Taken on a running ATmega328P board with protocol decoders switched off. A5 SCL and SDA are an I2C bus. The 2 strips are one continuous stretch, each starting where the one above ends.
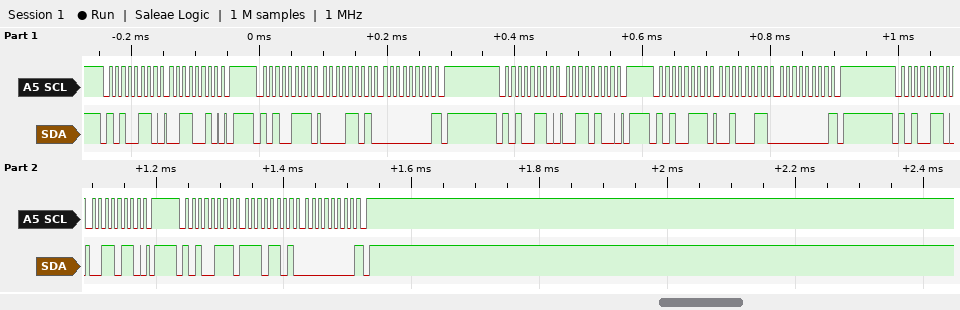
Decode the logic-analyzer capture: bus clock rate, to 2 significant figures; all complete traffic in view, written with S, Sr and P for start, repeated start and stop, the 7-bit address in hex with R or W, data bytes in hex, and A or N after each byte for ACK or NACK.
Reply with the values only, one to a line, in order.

100 kHz
S 53W A 32 A P S 53R A 0D A 00 N P S 53W A 34 A P S 53R A 23 A 00 N P S 53W A 36 A P S 53R A ED A 00 N P
